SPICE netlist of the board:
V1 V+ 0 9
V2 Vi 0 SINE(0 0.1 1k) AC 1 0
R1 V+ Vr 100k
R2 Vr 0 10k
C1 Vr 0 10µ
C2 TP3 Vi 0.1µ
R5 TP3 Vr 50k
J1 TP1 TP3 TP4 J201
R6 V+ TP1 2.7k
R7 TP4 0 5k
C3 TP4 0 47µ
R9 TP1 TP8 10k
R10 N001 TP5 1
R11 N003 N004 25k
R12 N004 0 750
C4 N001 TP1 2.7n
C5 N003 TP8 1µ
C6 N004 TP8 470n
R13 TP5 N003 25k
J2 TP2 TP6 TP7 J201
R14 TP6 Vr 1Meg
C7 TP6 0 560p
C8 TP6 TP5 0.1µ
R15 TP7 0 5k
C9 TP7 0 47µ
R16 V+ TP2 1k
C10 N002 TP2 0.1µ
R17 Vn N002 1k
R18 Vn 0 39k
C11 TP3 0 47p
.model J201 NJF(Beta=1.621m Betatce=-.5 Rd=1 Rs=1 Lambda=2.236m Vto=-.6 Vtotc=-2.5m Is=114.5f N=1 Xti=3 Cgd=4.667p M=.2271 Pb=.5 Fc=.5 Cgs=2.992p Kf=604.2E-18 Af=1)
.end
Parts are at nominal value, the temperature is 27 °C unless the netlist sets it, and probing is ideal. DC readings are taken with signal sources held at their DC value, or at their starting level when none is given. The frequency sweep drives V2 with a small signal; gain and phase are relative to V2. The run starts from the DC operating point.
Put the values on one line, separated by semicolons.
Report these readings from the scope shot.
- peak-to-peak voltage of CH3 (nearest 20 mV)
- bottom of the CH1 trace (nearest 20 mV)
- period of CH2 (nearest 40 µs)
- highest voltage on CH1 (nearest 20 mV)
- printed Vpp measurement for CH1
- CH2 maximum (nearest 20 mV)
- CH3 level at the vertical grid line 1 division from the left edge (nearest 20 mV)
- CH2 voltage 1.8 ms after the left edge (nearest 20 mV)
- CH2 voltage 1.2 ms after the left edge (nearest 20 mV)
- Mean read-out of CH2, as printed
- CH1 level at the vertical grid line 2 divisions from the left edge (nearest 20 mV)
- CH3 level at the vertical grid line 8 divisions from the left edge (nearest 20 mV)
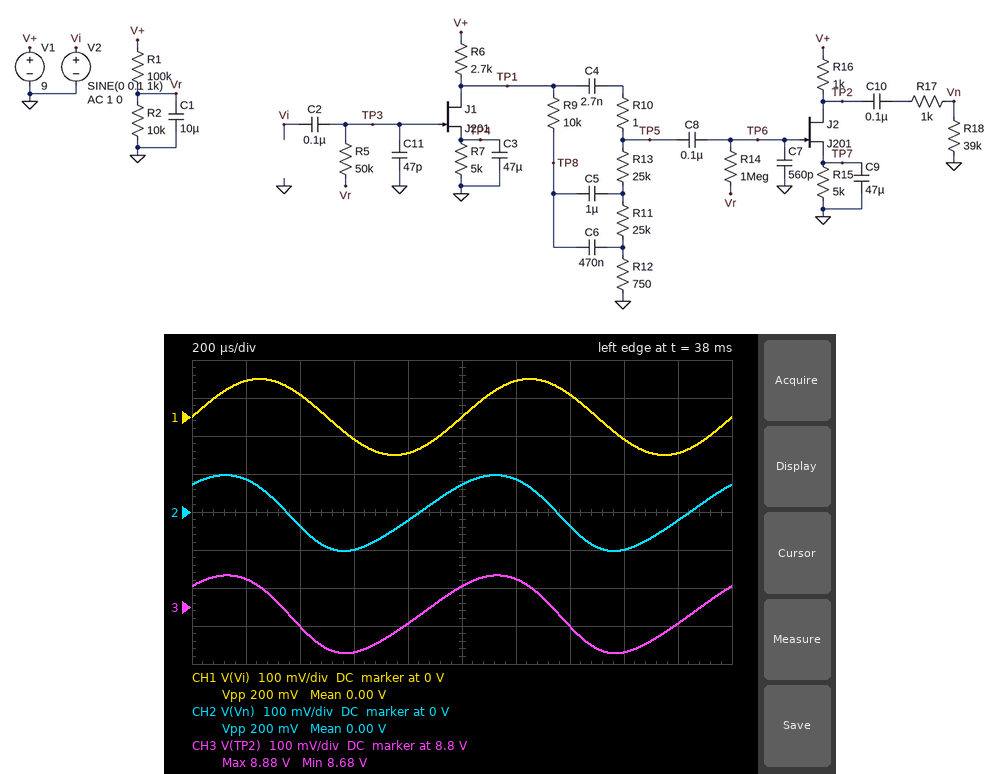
200 mV; -100 mV; 1.00 ms; 100 mV; 200 mV; 100 mV; 8.88 V; -20 mV; 80 mV; 0.00 V; 60 mV; 8.68 V
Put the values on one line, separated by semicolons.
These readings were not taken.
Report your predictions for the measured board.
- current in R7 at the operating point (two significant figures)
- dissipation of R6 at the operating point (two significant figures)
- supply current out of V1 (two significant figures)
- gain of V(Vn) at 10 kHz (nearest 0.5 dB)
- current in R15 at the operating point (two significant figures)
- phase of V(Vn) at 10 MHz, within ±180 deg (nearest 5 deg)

210 µA; 120 µW; 510 µA; 7.0 dB; 210 µA; -100 deg
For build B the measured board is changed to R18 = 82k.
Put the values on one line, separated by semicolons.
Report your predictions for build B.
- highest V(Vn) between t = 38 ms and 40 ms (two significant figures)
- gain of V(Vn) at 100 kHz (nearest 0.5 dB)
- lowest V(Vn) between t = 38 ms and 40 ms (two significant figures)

99 mV; 6.0 dB; -110 mV
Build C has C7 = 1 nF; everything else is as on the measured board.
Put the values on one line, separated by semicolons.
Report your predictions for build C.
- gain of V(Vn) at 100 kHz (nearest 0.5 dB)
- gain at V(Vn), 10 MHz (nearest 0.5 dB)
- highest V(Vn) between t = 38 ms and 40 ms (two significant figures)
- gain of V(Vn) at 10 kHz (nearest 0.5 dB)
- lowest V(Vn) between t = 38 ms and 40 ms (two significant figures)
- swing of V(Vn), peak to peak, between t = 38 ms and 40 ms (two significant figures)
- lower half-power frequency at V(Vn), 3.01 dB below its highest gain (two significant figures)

3.0 dB; -33.5 dB; 94 mV; 6.0 dB; -99 mV; 190 mV; 1.7 kHz
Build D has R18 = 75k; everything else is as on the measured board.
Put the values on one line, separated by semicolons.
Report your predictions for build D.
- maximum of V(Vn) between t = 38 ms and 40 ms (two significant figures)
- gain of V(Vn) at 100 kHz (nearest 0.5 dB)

99 mV; 6.0 dB
